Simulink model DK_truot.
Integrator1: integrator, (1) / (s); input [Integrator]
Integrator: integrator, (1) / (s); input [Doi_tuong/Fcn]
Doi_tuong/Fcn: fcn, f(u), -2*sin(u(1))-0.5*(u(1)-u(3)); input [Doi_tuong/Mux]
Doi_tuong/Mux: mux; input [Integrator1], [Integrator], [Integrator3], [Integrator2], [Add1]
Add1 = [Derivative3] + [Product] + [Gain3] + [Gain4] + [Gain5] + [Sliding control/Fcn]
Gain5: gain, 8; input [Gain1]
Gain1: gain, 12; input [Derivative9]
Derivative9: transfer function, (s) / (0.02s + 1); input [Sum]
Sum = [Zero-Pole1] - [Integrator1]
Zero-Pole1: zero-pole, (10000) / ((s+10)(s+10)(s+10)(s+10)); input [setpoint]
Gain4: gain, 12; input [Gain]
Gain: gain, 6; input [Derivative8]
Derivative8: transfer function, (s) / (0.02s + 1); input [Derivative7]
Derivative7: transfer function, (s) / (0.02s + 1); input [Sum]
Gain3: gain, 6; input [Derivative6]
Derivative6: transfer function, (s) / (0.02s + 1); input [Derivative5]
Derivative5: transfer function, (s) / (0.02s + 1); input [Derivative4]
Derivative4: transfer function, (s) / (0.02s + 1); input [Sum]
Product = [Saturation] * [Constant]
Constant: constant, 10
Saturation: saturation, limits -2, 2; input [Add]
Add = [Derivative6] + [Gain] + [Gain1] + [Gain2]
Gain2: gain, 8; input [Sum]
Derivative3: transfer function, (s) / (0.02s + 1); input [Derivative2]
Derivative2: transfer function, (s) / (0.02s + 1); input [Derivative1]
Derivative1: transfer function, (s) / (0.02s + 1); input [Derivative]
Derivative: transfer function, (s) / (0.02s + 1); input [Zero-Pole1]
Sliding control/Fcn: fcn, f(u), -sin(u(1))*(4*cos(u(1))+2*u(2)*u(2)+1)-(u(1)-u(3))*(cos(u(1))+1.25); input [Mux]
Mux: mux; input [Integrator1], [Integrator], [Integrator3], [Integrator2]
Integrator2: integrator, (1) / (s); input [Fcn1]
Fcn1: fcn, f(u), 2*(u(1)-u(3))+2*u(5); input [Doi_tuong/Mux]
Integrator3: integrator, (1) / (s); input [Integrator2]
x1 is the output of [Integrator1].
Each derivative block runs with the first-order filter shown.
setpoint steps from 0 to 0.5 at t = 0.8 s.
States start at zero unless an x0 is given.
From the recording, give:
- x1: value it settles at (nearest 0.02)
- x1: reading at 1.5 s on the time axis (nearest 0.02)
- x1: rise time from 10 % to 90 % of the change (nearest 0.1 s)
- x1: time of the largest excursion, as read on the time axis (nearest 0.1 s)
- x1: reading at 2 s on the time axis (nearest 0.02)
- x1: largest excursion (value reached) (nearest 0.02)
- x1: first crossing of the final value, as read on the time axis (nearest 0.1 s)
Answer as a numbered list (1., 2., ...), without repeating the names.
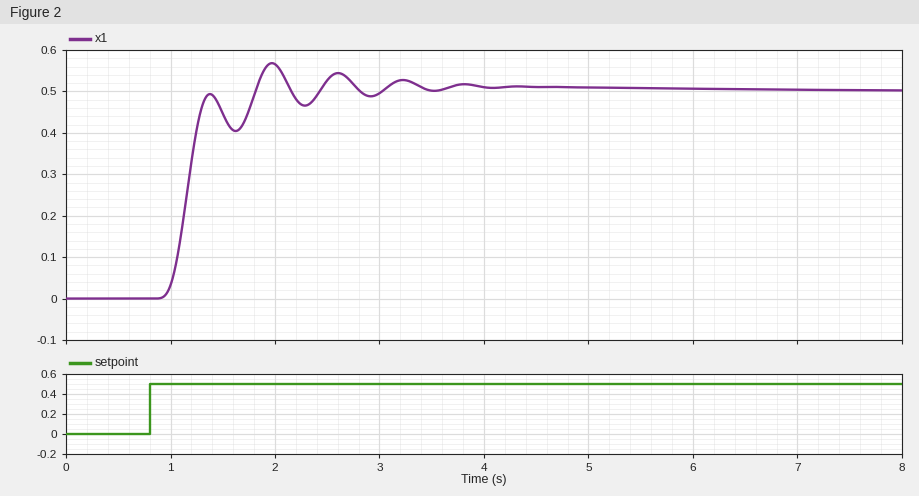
1. 0.50
2. 0.44
3. 0.3 s
4. 2.0 s
5. 0.56
6. 0.56
7. 1.8 s
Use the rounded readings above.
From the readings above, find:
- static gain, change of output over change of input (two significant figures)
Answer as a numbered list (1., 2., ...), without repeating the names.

1. 1.0
